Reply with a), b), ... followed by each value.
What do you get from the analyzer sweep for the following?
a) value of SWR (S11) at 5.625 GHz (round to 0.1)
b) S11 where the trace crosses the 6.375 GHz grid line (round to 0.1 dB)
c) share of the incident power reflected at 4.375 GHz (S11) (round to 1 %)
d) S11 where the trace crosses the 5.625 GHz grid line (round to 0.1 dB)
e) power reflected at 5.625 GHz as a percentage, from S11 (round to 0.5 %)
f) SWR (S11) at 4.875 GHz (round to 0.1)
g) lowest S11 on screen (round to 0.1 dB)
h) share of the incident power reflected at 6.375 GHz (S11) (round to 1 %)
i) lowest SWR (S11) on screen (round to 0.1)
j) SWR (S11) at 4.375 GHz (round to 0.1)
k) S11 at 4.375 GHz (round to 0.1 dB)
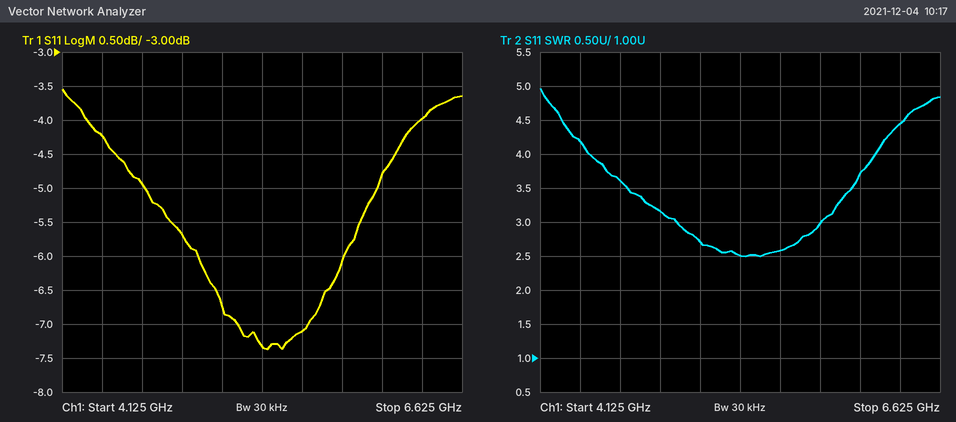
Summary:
a) 2.6
b) -4.0 dB
c) 38 %
d) -7.1 dB
e) 19.5 %
f) 3.2
g) -7.4 dB
h) 40 %
i) 2.5
j) 4.2
k) -4.2 dB
